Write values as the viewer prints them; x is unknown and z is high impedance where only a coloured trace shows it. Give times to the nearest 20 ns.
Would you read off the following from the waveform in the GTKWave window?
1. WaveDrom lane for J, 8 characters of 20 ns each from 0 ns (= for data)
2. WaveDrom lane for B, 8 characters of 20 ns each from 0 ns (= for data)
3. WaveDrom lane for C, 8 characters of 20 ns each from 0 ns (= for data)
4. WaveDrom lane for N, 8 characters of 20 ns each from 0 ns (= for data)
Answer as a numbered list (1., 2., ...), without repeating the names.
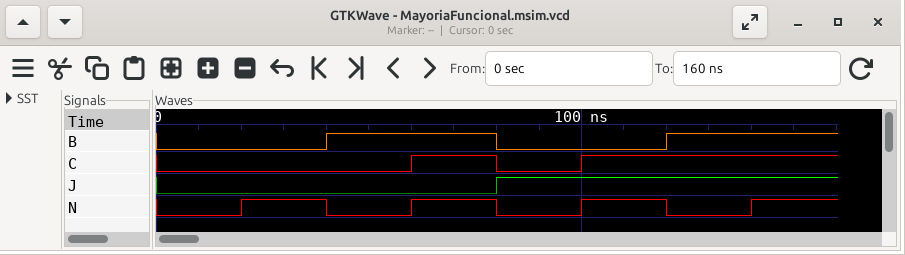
1. {name: 'J', wave: '0...1...'}
2. {name: 'B', wave: '0.1.0.1.'}
3. {name: 'C', wave: '0..101..'}
4. {name: 'N', wave: '01010101'}
